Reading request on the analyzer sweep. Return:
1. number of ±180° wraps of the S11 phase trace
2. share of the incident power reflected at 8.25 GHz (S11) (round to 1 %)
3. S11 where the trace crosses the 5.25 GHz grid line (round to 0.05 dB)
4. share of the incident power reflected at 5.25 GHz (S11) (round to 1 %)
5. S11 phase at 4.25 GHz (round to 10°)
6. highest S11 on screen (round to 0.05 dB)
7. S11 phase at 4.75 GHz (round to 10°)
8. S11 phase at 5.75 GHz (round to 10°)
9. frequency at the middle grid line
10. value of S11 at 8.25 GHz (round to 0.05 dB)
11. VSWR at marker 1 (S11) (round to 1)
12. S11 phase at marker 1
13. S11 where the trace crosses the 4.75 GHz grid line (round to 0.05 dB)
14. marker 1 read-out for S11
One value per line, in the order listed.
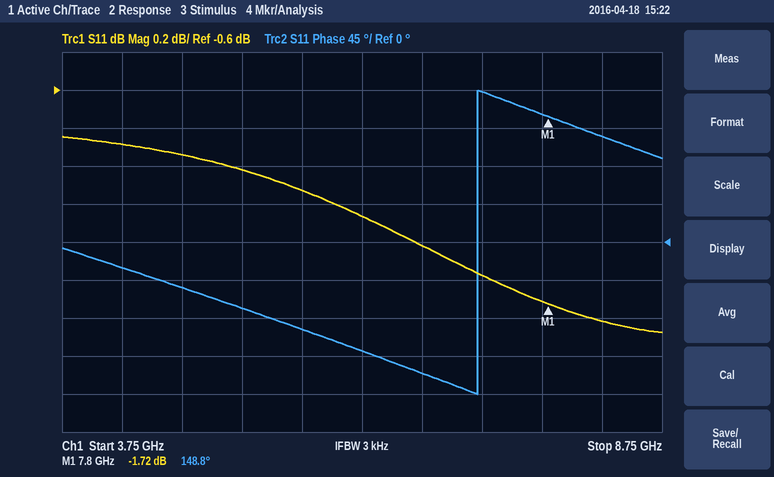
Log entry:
1
66 %
-1.00 dB
79 %
-30°
-0.85 dB
-50°
-100°
6.25 GHz
-1.80 dB
10
148.8°
-0.95 dB
-1.72 dB
